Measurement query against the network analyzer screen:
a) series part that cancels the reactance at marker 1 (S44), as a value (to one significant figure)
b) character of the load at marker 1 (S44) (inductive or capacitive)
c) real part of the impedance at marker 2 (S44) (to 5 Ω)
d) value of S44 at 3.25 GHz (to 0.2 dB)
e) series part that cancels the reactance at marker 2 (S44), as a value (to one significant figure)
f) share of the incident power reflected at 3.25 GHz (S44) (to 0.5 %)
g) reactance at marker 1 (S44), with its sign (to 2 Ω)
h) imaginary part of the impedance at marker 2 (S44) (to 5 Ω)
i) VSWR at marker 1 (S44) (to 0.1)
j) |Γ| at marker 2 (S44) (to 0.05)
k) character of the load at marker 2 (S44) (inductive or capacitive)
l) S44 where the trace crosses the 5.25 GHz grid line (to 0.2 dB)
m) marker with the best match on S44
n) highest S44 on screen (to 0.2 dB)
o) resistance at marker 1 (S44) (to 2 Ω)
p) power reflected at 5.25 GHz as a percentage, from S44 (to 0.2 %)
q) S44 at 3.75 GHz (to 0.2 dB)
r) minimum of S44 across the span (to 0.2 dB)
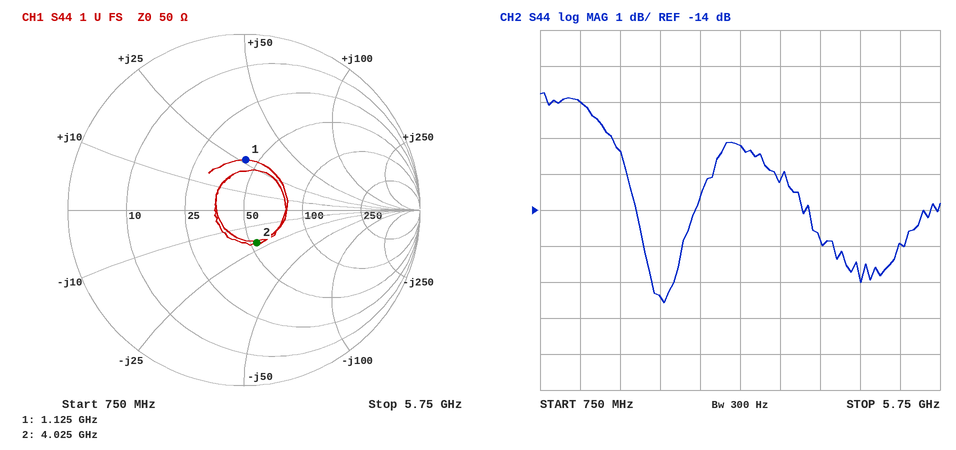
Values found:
5 pF
inductive
55 Ω
-12.2 dB
800 pH
6.0 %
+26 Ω
-20 Ω
1.8
0.20
capacitive
-15.0 dB
marker 2
-10.8 dB
44 Ω
3.2 %
-13.2 dB
-16.6 dB
